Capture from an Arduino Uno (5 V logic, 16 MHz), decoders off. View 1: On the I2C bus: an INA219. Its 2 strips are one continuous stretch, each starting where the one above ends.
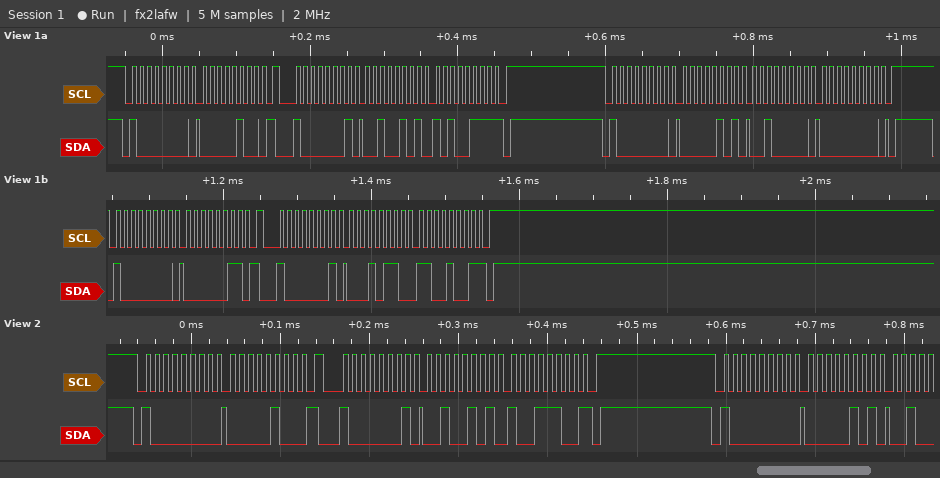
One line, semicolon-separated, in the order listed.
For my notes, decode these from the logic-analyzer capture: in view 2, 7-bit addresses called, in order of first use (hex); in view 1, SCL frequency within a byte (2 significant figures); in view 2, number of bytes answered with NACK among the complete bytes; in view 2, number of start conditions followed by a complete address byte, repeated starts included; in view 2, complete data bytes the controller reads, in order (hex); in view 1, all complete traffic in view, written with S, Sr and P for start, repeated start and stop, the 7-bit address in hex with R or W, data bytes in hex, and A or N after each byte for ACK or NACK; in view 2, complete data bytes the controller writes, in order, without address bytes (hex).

0x40; 100 kHz; 1; 3; 25 9C; S 40W A 04 A Sr 40R A 25 A A7 N P S 40W A 05 A 20 A 00 A P S 40W A 03 A Sr 40R A 16 A C9 N P; 04 05
